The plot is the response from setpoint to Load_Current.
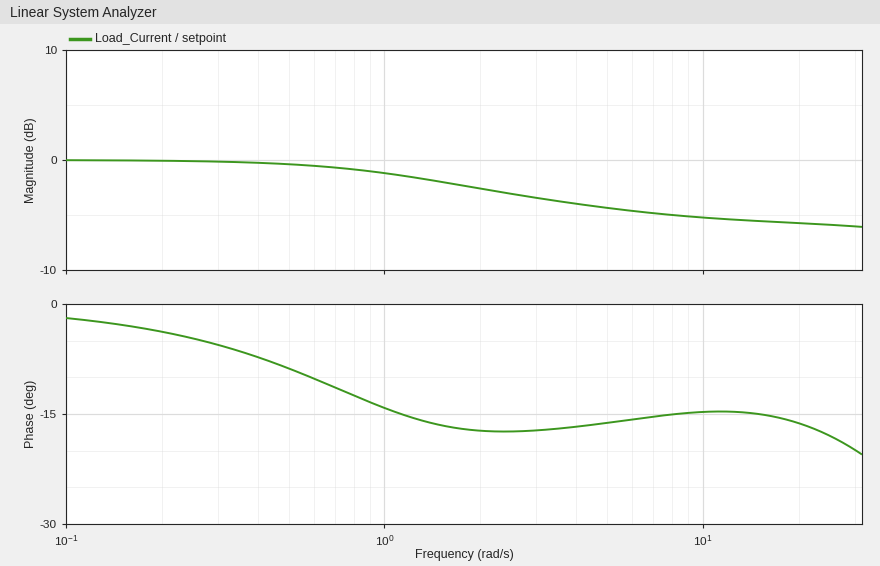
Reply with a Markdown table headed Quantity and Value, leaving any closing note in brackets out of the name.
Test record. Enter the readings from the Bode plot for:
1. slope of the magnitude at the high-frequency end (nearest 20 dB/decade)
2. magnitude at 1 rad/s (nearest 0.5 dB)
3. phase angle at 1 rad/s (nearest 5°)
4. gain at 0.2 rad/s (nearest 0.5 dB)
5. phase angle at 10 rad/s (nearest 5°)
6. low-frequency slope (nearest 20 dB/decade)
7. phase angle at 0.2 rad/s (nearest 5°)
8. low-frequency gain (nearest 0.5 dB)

| Quantity | Value |
|---|---|
| slope of the magnitude at the high-frequency end | 0 dB/decade |
| magnitude at 1 rad/s | -1.0 dB |
| phase angle at 1 rad/s | -15° |
| gain at 0.2 rad/s | 0.0 dB |
| phase angle at 10 rad/s | -15° |
| low-frequency slope | 0 dB/decade |
| phase angle at 0.2 rad/s | -5° |
| low-frequency gain | 0.0 dB |
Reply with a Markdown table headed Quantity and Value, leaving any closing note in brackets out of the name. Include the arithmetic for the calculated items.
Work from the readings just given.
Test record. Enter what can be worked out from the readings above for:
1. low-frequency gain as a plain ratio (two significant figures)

| Quantity | Value |
|---|---|
| low-frequency gain as a plain ratio | 10^(0 / 20) = 1.0 |
